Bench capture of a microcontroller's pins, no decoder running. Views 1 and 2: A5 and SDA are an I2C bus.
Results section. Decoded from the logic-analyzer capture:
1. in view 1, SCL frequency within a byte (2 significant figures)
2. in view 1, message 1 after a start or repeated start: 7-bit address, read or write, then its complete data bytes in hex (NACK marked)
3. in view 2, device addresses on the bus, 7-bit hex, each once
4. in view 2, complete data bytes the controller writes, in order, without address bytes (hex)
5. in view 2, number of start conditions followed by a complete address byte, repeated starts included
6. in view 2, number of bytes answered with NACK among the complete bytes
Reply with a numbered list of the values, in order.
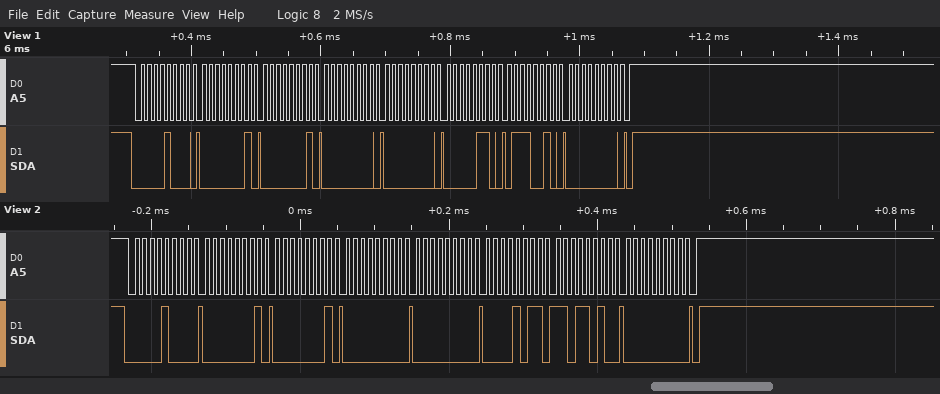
1. 100 kHz
2. 0x04 write: 01 01 00 00 06 72 00
3. 0x04
4. 01 01 00 00 0B DA 00
5. 1
6. 0
